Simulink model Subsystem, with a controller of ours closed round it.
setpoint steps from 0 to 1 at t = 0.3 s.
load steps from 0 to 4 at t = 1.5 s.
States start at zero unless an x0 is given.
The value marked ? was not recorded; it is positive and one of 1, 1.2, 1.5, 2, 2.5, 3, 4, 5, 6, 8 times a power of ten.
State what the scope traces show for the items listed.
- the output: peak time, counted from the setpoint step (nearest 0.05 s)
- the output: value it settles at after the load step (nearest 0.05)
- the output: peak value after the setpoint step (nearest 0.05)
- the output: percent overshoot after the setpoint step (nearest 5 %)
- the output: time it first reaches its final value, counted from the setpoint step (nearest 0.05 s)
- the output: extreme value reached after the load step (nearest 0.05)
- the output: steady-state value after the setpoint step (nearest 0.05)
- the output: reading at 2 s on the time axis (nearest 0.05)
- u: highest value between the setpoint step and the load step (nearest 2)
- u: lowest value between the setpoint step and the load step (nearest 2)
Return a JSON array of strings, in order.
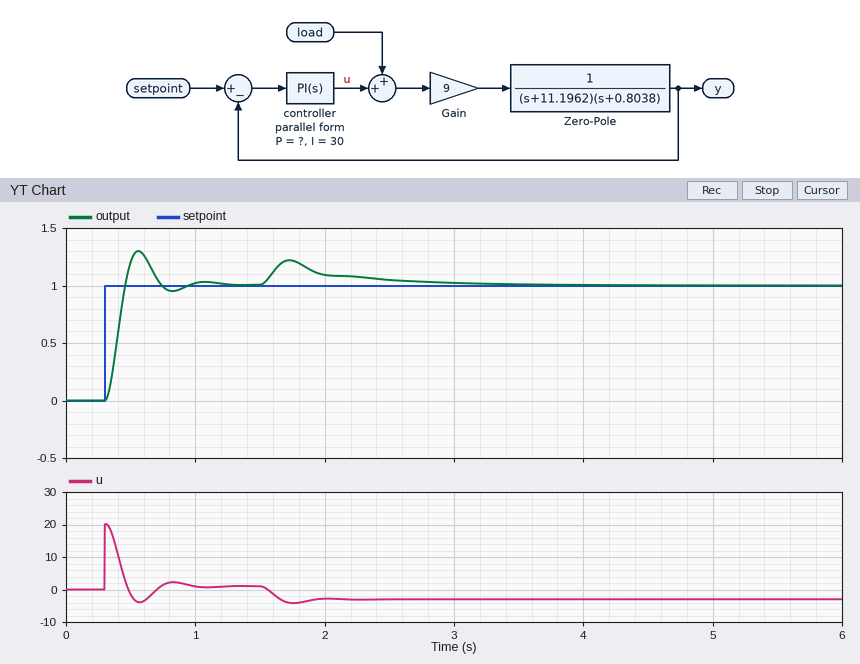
["0.25 s", "1.00", "1.30", "30 %", "0.15 s", "1.20", "1.00", "1.10", "20", "-4"]
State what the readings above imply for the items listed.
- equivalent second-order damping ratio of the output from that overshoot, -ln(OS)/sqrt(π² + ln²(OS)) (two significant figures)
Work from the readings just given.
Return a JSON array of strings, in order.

["0.36"]
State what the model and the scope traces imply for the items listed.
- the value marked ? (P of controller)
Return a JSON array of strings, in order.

["20"]
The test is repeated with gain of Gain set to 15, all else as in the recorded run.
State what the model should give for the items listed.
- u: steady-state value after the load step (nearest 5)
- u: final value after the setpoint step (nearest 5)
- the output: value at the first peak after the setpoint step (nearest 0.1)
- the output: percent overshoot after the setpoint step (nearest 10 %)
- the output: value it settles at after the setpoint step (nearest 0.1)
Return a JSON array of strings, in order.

["-5", "0", "1.4", "40 %", "1.0"]
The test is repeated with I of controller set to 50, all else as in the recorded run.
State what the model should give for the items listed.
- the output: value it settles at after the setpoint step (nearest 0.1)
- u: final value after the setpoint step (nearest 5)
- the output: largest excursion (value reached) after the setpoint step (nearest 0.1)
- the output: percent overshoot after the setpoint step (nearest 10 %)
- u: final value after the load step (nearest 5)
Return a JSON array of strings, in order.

["1.0", "0", "1.4", "40 %", "-5"]
